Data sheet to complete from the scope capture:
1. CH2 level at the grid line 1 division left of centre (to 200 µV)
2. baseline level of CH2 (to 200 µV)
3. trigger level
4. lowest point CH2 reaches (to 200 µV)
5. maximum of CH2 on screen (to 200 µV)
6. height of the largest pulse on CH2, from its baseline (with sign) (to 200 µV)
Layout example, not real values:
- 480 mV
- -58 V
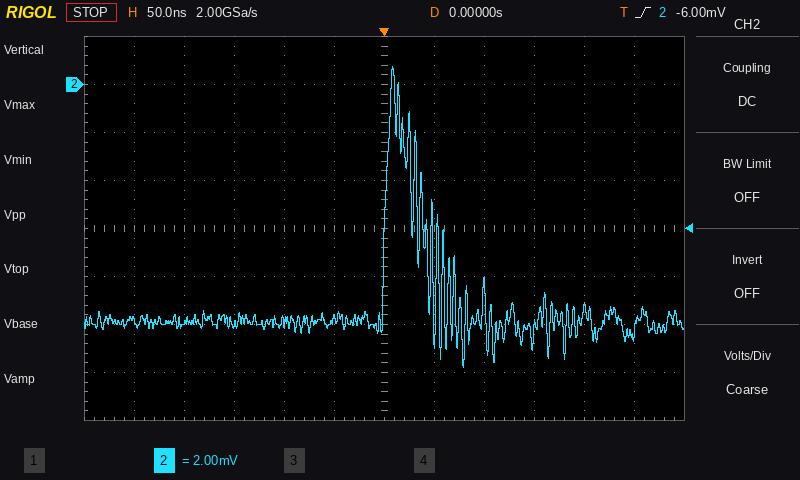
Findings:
- -9.8 mV
- -9.8 mV
- -6.00 mV
- -11.8 mV
- 800 µV
- +10.6 mV
